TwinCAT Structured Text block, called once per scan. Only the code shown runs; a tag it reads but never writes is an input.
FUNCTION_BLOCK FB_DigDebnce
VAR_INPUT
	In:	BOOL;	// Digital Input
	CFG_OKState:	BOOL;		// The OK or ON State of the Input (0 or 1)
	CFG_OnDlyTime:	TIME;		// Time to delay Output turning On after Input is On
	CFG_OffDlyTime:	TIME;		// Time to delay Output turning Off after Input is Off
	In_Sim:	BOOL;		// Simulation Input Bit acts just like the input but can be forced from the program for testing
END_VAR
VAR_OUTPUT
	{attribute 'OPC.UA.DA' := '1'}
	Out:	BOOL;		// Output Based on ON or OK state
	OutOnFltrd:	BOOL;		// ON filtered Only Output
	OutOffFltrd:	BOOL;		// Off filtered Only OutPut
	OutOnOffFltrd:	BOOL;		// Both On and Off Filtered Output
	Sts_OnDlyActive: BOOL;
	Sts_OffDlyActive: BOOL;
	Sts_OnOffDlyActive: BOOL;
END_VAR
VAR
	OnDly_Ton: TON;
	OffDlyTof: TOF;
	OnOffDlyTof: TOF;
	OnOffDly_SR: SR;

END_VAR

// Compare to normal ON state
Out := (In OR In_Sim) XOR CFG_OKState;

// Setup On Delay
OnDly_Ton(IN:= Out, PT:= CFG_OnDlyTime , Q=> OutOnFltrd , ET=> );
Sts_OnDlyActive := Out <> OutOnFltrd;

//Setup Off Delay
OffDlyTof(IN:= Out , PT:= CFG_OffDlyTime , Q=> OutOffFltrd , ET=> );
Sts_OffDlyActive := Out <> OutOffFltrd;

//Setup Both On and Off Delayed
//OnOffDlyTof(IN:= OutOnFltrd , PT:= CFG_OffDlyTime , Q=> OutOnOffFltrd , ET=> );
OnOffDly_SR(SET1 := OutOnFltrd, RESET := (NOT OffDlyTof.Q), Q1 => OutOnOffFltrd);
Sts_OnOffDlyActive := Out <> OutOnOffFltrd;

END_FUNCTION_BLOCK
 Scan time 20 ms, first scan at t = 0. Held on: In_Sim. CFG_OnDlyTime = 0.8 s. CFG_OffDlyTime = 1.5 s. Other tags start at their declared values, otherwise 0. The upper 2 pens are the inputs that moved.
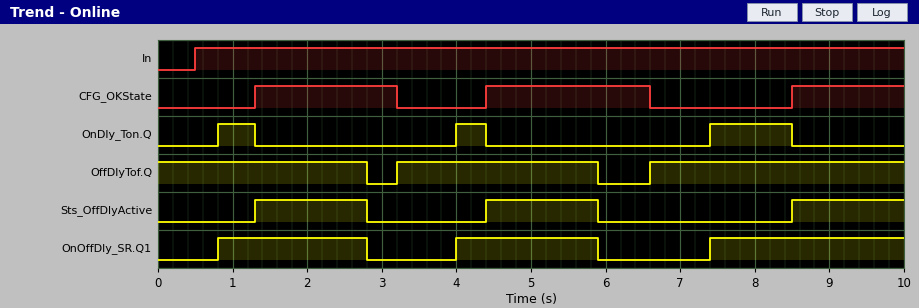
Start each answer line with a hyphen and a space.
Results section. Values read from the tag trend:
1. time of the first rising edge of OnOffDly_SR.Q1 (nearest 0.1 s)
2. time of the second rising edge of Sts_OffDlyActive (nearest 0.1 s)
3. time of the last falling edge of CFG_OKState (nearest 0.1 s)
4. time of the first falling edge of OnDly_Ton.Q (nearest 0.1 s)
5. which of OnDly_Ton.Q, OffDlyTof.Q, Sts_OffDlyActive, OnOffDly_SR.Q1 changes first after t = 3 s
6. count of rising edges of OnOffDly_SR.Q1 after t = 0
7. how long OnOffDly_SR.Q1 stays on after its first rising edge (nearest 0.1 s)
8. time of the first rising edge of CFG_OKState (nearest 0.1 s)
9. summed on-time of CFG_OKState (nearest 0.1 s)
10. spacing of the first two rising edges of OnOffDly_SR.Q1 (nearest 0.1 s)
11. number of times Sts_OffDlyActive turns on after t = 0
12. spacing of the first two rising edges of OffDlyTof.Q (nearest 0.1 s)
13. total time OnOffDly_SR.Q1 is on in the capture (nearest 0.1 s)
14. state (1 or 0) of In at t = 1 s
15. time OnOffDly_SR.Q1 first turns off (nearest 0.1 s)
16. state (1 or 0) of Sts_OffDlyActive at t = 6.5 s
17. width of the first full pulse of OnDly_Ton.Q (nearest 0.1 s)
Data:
- 0.8 s
- 4.4 s
- 6.6 s
- 1.3 s
- OffDlyTof.Q
- 3
- 2.0 s
- 1.3 s
- 5.6 s
- 3.2 s
- 3
- 3.4 s
- 6.5 s
- 1
- 2.8 s
- 0
- 0.5 s
